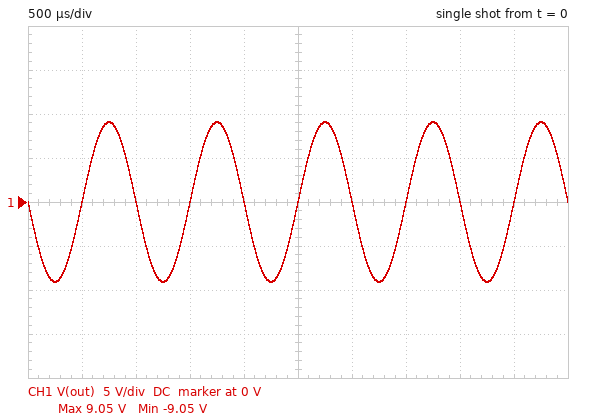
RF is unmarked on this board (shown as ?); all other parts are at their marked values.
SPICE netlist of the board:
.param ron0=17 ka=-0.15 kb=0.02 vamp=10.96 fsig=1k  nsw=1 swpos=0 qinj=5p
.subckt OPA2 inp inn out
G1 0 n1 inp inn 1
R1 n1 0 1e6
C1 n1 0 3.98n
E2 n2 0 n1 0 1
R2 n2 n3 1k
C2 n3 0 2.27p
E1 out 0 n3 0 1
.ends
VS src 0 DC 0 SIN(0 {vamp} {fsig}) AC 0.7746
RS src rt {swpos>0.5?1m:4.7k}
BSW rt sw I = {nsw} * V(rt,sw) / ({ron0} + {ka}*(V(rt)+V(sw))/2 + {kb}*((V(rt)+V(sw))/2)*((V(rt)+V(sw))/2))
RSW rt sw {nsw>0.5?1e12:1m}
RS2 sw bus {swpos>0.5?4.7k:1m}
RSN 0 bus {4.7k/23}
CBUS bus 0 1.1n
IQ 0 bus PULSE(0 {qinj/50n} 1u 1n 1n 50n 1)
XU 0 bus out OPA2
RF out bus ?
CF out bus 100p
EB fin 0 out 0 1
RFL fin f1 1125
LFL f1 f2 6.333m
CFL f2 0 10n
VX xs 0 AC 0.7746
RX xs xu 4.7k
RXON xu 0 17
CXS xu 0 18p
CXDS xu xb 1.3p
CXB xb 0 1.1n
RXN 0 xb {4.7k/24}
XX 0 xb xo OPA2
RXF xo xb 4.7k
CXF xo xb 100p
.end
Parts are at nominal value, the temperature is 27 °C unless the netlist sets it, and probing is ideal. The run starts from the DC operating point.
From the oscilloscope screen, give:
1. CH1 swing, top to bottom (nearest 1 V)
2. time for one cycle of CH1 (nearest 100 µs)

18 V
1.0 ms
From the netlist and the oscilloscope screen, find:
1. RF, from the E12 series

3.9 kΩ
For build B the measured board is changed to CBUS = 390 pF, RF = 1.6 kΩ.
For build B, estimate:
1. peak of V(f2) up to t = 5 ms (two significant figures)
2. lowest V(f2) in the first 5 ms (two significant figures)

3.7 V
-3.7 V
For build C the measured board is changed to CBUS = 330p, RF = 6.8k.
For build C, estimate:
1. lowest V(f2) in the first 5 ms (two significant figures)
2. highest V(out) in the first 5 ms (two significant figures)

-16 V
16 V
